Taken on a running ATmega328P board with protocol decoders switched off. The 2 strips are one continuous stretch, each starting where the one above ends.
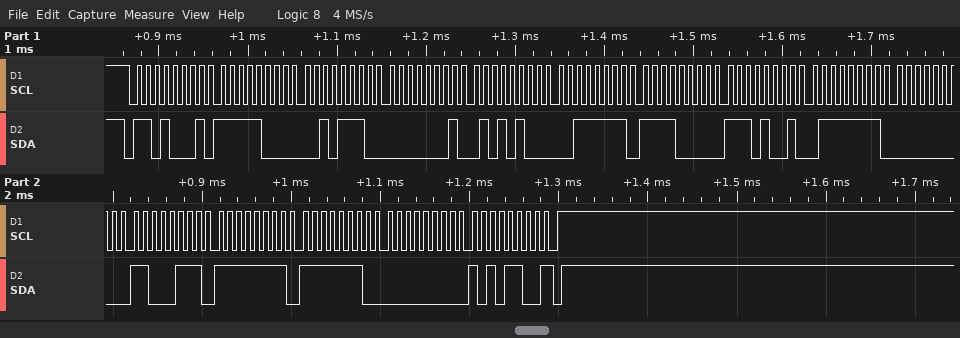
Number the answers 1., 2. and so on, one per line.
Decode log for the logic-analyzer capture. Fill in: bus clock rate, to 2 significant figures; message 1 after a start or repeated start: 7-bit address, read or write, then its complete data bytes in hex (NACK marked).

1. 100 kHz
2. 0x68 read: F8 2E 01 54 3F F0 E9 7F 00 C7 FF FE 00 AC NACK
